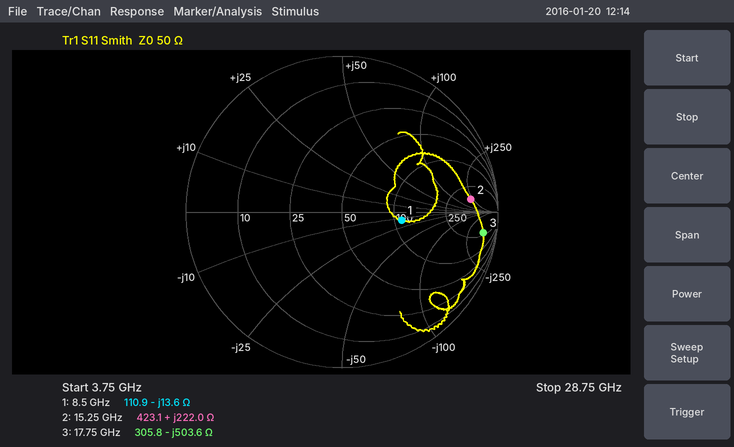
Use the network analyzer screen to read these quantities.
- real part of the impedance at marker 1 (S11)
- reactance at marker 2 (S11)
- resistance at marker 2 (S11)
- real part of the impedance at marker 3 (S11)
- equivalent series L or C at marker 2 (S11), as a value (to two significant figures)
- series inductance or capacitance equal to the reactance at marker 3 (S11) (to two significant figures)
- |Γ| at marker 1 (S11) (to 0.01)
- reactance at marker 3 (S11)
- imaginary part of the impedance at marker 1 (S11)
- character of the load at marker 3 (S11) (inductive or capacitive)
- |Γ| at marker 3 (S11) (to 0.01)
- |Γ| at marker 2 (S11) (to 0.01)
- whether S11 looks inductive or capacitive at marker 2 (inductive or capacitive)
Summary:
110.9 Ω
+222.0 Ω
423.1 Ω
305.8 Ω
2.3 nH
18 fF
0.39
-503.6 Ω
-13.6 Ω
capacitive
0.92
0.83
inductive
